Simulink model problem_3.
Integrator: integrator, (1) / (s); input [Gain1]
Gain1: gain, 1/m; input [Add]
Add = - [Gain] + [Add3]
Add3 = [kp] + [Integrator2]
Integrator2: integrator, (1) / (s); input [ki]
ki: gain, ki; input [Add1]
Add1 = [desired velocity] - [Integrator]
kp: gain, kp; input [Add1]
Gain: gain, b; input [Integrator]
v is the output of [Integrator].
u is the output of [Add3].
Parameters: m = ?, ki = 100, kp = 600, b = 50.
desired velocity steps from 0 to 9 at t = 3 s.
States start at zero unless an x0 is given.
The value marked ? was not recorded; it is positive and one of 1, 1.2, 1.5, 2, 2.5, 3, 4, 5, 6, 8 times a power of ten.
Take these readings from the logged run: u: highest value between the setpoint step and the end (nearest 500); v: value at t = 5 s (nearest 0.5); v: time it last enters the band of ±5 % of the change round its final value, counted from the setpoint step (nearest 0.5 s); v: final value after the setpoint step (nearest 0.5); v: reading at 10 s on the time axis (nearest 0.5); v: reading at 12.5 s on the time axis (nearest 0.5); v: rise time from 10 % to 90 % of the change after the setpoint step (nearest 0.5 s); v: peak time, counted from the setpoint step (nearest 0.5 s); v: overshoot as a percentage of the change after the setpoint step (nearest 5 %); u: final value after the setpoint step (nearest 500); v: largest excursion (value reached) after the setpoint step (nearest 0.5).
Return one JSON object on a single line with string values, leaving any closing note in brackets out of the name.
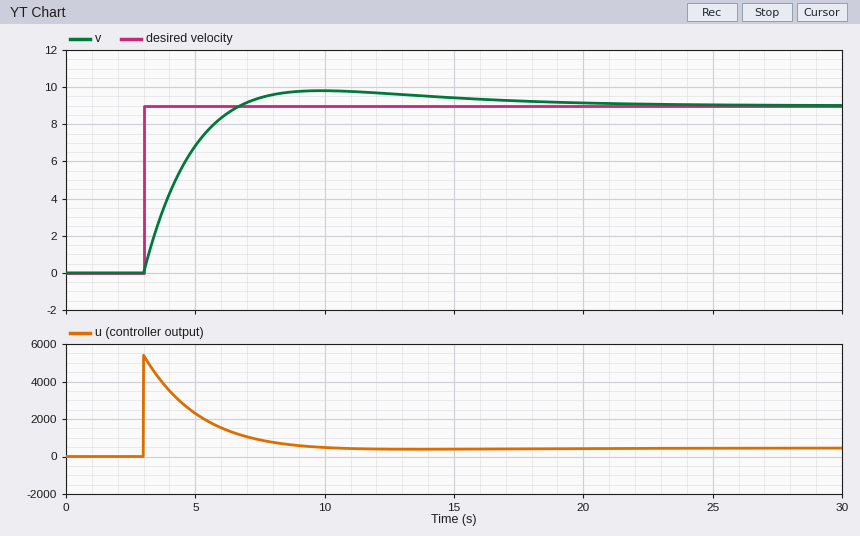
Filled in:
{"u: highest value between the setpoint step and the end": "5500", "v: value at t = 5 s": "7.0", "v: time it last enters the band of ±5 % of the change round its final value, counted from the setpoint step": "11.5 s", "v: final value after the setpoint step": "9.0", "v: reading at 10 s on the time axis": "10.0", "v: reading at 12.5 s on the time axis": "9.5", "v: rise time from 10 % to 90 % of the change after the setpoint step": "2.5 s", "v: peak time, counted from the setpoint step": "7.0 s", "v: overshoot as a percentage of the change after the setpoint step": "10 %", "u: final value after the setpoint step": "500", "v: largest excursion (value reached) after the setpoint step": "10.0"}
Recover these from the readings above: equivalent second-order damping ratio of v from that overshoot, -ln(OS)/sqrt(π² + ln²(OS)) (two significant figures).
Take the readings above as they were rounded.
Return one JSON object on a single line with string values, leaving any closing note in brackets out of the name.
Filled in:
{"equivalent second-order damping ratio of v from that overshoot, -ln(OS)/sqrt(π² + ln²(OS))": "0.59"}
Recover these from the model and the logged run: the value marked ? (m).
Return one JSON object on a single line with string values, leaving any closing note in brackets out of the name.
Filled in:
{"the value marked ?": "1000"}
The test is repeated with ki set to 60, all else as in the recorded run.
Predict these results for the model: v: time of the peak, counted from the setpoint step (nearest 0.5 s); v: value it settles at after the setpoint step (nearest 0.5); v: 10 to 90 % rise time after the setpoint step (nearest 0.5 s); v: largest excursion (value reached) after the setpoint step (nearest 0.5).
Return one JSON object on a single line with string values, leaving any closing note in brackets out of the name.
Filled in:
{"v: time of the peak, counted from the setpoint step": "8.5 s", "v: value it settles at after the setpoint step": "9.0", "v: 10 to 90 % rise time after the setpoint step": "3.0 s", "v: largest excursion (value reached) after the setpoint step": "9.5"}
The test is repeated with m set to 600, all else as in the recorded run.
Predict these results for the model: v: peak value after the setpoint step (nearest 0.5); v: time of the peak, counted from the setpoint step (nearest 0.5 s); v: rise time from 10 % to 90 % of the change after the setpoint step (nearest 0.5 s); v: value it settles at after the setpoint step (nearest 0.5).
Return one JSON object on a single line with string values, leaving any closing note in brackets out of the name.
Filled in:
{"v: peak value after the setpoint step": "9.5", "v: time of the peak, counted from the setpoint step": "5.0 s", "v: rise time from 10 % to 90 % of the change after the setpoint step": "2.0 s", "v: value it settles at after the setpoint step": "9.0"}
